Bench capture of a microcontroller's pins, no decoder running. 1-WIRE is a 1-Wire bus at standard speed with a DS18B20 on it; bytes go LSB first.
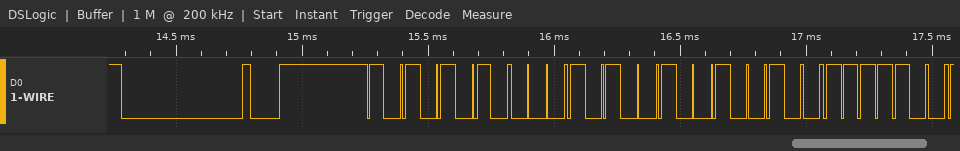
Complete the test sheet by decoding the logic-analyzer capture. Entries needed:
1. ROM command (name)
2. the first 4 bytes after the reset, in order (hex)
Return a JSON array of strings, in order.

["Match ROM", "55 28 49 3E"]
